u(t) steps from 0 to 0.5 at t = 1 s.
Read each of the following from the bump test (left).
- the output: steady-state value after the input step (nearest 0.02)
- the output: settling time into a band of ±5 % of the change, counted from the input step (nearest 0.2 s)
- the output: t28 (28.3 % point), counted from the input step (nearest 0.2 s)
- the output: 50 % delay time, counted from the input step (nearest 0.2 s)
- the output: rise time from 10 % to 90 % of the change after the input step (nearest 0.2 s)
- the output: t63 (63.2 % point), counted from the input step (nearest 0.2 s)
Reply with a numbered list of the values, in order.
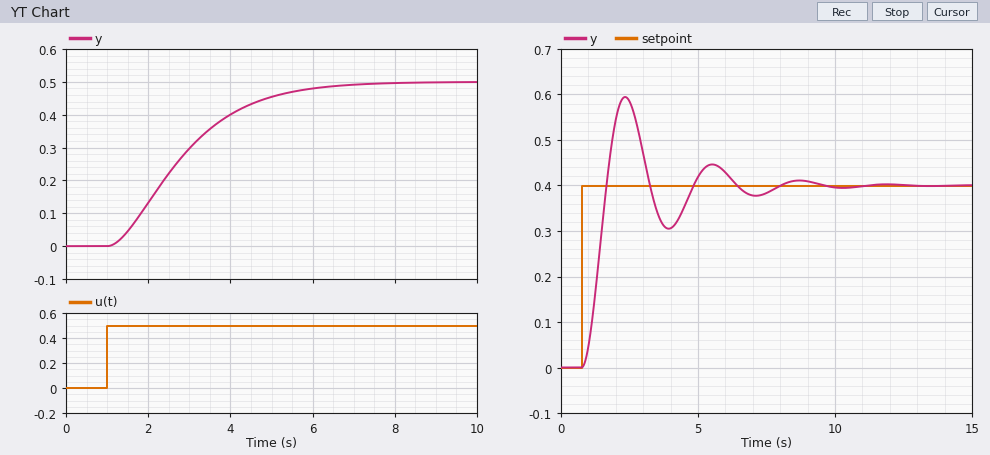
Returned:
1. 0.50
2. 4.8 s
3. 1.0 s
4. 1.6 s
5. 3.4 s
6. 2.2 s
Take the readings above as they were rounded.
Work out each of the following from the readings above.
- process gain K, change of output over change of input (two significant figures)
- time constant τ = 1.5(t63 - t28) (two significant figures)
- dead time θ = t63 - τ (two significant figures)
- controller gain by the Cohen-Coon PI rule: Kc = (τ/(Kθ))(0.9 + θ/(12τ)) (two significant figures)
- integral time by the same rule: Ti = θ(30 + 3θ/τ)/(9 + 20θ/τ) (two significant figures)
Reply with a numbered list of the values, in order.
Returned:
1. 1.0
2. 1.8 s
3. 0.40 s
4. 4.1
5. 0.91 s
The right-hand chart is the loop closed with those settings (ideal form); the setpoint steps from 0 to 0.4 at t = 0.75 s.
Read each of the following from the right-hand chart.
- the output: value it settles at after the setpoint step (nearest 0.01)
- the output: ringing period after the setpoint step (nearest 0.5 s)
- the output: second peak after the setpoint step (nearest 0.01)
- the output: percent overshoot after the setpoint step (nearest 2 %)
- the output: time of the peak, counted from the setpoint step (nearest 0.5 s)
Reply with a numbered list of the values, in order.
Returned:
1. 0.40
2. 3.0 s
3. 0.45
4. 48 %
5. 1.5 s
